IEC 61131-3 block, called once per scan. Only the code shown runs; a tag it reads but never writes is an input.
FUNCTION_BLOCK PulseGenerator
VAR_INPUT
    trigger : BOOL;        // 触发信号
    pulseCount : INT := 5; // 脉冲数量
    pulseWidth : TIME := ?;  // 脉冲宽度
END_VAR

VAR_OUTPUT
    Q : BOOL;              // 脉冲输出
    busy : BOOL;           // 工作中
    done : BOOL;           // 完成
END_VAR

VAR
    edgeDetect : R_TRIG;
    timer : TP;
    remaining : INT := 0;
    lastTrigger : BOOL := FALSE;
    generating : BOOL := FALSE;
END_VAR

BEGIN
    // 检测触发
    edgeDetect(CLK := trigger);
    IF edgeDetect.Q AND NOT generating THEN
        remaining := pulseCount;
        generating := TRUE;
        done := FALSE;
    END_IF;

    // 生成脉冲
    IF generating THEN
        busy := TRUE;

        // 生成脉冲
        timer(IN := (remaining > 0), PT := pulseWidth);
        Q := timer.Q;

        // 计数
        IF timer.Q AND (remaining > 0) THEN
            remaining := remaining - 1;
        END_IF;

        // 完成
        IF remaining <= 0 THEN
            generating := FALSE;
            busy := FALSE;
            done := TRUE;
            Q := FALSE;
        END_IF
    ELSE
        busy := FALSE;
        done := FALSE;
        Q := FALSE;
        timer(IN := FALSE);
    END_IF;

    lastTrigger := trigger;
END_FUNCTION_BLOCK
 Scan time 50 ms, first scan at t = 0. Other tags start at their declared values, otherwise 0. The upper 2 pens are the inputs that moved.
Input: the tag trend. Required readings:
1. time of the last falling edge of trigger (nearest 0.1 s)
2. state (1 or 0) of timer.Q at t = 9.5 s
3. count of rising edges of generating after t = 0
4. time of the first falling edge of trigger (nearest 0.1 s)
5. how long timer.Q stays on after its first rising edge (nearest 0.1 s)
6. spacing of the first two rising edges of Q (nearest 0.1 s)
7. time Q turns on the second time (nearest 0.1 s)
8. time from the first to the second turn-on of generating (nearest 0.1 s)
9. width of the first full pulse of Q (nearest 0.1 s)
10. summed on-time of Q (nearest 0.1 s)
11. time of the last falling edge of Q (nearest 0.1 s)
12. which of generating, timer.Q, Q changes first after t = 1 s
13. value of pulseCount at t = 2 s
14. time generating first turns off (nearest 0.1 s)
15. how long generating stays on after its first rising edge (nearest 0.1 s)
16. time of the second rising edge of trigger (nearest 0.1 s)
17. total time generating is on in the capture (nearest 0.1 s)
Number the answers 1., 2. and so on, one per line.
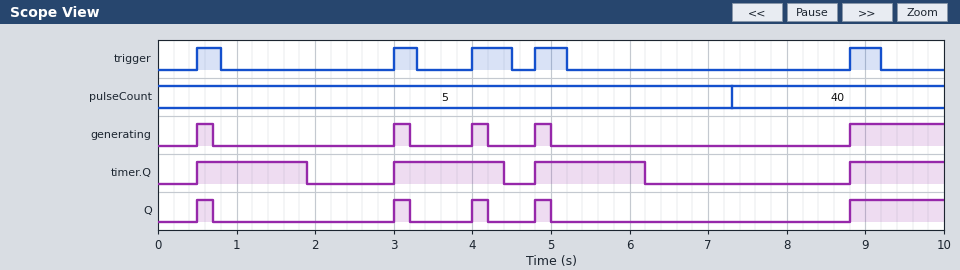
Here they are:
1. 9.2 s
2. 1
3. 5
4. 0.8 s
5. 1.4 s
6. 2.5 s
7. 3.0 s
8. 2.5 s
9. 0.2 s
10. 2.0 s
11. 5.0 s
12. timer.Q
13. 5
14. 0.7 s
15. 0.2 s
16. 3.0 s
17. 2.0 s
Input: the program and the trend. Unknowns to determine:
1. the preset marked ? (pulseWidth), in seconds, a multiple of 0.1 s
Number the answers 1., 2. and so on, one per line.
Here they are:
1. 1.4 s
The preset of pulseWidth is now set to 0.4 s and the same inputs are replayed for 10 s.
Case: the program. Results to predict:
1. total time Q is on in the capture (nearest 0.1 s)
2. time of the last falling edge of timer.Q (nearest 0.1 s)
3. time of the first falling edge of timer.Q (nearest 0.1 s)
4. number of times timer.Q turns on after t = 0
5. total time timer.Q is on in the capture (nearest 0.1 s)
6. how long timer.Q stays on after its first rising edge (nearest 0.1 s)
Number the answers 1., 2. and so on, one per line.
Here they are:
1. 1.2 s
2. 9.2 s
3. 0.9 s
4. 5
5. 2.0 s
6. 0.4 s
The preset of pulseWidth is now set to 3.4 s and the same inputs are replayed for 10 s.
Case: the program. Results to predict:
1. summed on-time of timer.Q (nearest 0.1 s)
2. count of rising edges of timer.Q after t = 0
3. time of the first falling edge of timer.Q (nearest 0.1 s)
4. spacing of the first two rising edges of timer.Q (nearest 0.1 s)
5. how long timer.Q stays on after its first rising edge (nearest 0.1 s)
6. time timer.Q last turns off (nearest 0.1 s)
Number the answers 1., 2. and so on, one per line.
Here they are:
1. 8.0 s
2. 3
3. 3.9 s
4. 3.5 s
5. 3.4 s
6. 7.4 s
